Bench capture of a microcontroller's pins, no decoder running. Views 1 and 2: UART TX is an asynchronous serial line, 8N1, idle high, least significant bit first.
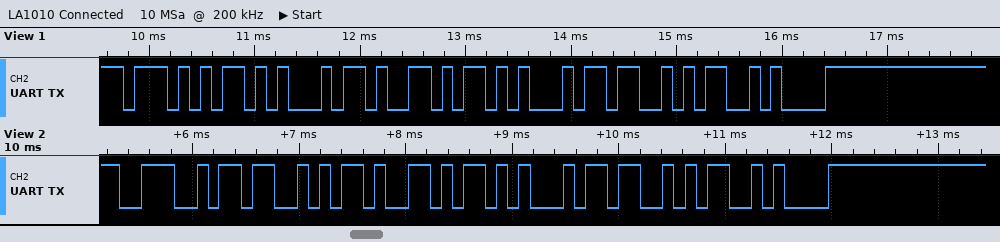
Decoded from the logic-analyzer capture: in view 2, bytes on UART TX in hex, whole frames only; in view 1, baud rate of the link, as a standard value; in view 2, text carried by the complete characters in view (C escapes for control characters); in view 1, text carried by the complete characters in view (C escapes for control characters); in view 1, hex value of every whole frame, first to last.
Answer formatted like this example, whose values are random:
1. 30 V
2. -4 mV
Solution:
1. 4E 53 59 45 53 0A
2. 9600 baud
3. "NSYES\n"
4. "WEYES\n"
5. 57 45 59 45 53 0A
